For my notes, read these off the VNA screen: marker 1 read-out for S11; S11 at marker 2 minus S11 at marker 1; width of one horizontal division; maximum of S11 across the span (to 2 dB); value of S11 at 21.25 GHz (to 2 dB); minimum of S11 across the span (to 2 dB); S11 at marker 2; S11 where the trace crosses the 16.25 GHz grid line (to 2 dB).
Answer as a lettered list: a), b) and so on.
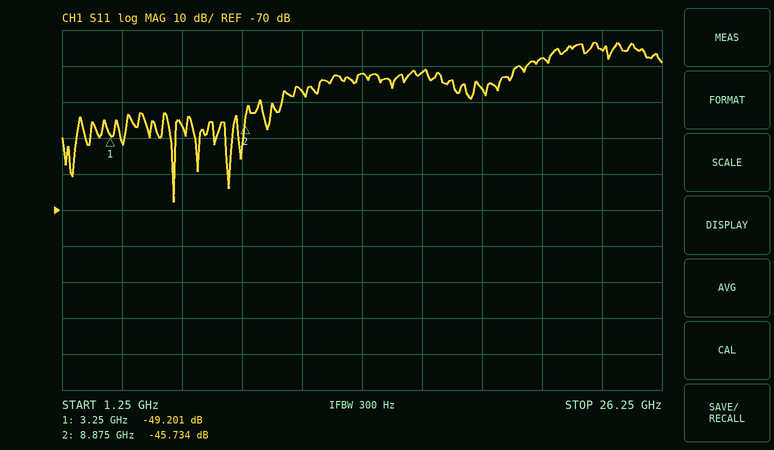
a) -49.201 dB
b) 3.467 dB
c) 2.5 GHz
d) -24 dB
e) -28 dB
f) -68 dB
g) -45.734 dB
h) -32 dB
